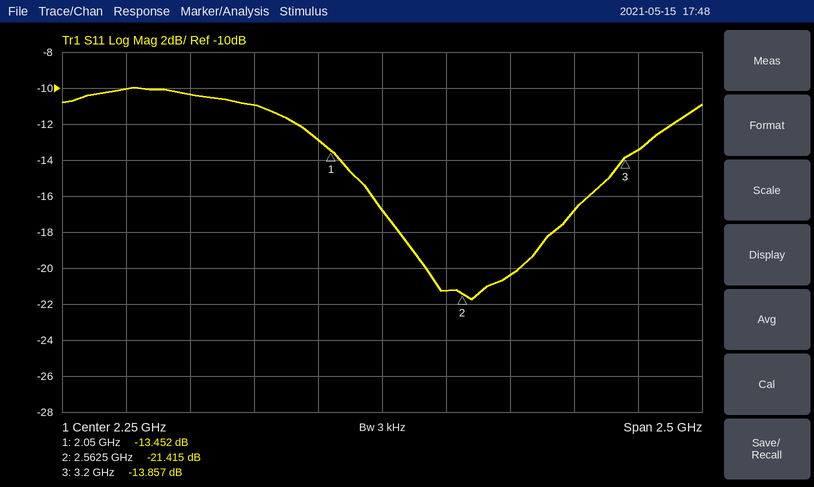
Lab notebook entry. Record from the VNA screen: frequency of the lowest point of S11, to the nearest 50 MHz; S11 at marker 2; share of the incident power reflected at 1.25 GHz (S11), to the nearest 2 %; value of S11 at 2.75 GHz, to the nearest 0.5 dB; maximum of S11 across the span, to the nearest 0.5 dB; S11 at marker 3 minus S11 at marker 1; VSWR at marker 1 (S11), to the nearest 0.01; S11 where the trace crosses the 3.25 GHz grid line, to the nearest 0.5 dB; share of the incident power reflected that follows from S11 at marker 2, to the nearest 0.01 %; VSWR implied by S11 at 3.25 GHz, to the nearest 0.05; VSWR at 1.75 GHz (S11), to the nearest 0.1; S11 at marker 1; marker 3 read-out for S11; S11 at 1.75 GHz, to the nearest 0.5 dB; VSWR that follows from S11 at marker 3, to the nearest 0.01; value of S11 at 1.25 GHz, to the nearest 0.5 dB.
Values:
2.60 GHz
-21.415 dB
10 %
-20.5 dB
-10.0 dB
-0.405 dB
1.54
-13.5 dB
0.72 %
1.55
1.8
-13.452 dB
-13.857 dB
-11.0 dB
1.51
-10.0 dB
